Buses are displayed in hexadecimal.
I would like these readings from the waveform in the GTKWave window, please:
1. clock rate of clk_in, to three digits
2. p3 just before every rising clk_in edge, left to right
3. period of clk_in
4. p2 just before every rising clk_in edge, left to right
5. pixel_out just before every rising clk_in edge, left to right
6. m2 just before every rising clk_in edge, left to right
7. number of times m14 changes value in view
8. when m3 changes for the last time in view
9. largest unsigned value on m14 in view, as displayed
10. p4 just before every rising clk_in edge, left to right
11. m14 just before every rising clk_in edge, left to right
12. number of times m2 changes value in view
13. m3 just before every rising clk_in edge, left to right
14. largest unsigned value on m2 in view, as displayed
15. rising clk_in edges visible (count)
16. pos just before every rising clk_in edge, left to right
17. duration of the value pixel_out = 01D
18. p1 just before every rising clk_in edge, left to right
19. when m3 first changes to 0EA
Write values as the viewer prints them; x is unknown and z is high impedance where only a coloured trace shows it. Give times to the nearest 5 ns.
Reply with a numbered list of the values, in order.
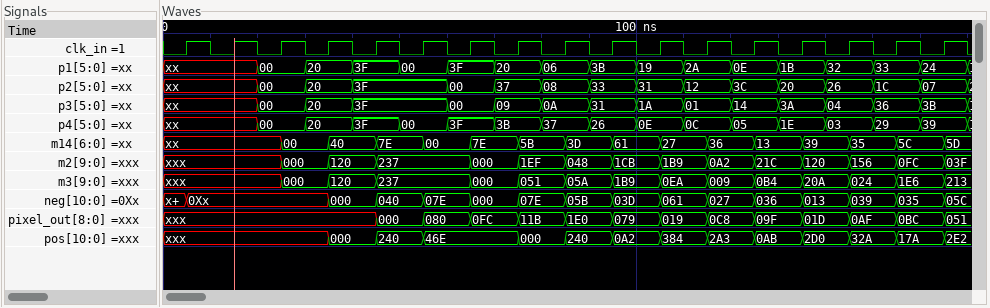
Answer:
1. 100 MHz
2. xx, xx, 00, 20, 3F, 3F, 00, 09, 0A, 31, 1A, 01, 14, 3A, 04, 36, 3B
3. 10 ns
4. xx, xx, 00, 20, 3F, 3F, 00, 37, 08, 33, 31, 12, 3C, 20, 26, 1C, 07
5. xxx, xxx, xxx, xxx, xxx, 000, 080, 0FC, 11B, 1E0, 079, 019, 0C8, 09F, 01D, 0AF, 0BC
6. xxx, xxx, xxx, 000, 120, 237, 237, 000, 1EF, 048, 1CB, 1B9, 0A2, 21C, 120, 156, 0FC
7. 15
8. 165 ns
9. 7E
10. xx, xx, 00, 20, 3F, 00, 3F, 3B, 37, 26, 0E, 0C, 05, 1E, 03, 29, 39
11. xx, xx, xx, 00, 40, 7E, 00, 7E, 5B, 3D, 61, 27, 36, 13, 39, 35, 5C
12. 14
13. xxx, xxx, xxx, 000, 120, 237, 237, 000, 051, 05A, 1B9, 0EA, 009, 0B4, 20A, 024, 1E6
14. 237
15. 17
16. xxx, xxx, xxx, xxx, 000, 240, 46E, 46E, 000, 240, 0A2, 384, 2A3, 0AB, 2D0, 32A, 17A
17. 10 ns
18. xx, xx, 00, 20, 3F, 00, 3F, 20, 06, 3B, 19, 2A, 0E, 1B, 32, 33, 24
19. 105 ns
